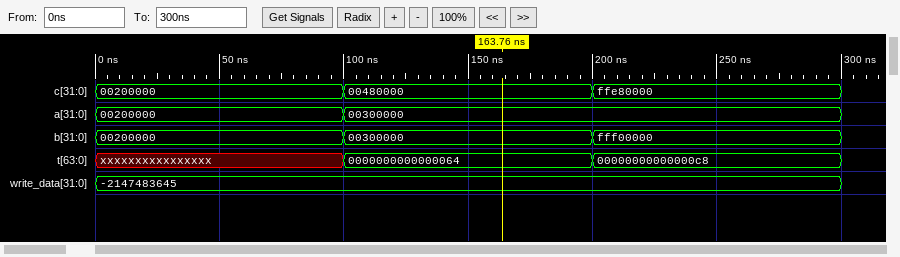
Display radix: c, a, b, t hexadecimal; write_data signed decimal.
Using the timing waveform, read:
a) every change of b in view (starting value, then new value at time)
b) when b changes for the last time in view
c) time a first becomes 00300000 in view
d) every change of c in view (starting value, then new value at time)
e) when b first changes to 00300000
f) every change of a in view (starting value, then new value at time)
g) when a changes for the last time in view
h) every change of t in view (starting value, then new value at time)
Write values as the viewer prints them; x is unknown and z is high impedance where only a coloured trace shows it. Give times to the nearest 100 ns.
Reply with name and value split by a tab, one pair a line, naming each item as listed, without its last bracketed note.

every change of b in view	00200000, 00300000 at 100 ns, fff00000 at 200 ns
when b changes for the last time in view	200 ns
time a first becomes 00300000 in view	100 ns
every change of c in view	00200000, 00480000 at 100 ns, ffe80000 at 200 ns
when b first changes to 00300000	100 ns
every change of a in view	00200000, 00300000 at 100 ns
when a changes for the last time in view	100 ns
every change of t in view	xxxxxxxxxxxxxxxx, 0000000000000064 at 100 ns, 00000000000000c8 at 200 ns
